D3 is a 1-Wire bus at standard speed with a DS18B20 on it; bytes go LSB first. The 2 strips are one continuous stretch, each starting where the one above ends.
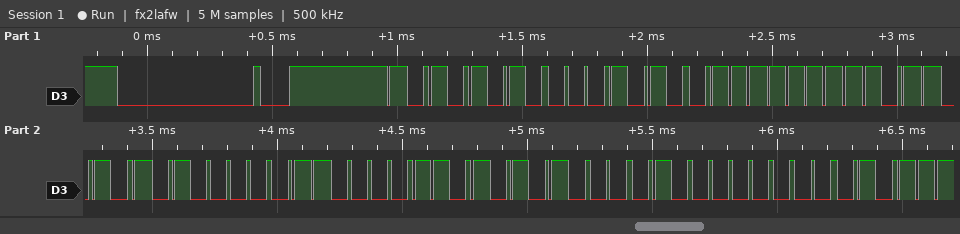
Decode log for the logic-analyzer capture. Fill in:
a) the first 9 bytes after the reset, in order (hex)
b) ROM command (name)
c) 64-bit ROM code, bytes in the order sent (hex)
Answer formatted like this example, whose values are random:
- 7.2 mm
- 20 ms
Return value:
- 55 28 FF AD 82 61 15 02 E8
- Match ROM
- 28 FF AD 82 61 15 02 E8
